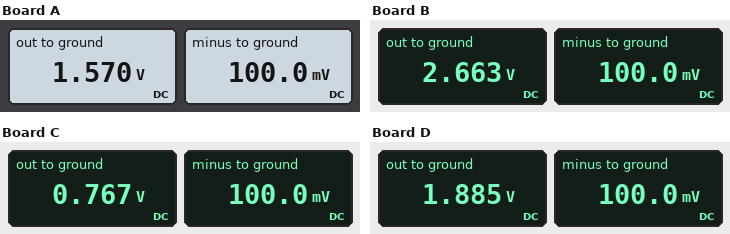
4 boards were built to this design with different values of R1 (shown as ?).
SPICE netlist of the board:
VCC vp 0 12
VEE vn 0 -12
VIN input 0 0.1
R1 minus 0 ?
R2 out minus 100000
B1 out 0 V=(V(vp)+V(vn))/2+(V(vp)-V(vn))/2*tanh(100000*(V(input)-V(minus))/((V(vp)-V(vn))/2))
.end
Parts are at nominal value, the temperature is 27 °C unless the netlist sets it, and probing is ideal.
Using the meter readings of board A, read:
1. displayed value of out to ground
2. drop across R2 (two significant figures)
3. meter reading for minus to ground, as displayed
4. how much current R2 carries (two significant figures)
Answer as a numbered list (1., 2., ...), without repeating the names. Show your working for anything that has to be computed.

1. 1.570 V
2. 1.57 V - 100 mV = 1.5 V
3. 100.0 mV
4. (1.57 V - 100 mV) / 100 kΩ = 15 µA
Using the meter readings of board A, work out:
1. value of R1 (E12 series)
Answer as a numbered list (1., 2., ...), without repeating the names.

1. 6.8 kΩ
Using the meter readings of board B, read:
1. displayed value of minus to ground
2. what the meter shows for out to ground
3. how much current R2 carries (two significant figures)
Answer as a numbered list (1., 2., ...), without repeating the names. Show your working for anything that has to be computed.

1. 100.0 mV
2. 2.663 V
3. (2.663 V - 100 mV) / 100 kΩ = 26 µA
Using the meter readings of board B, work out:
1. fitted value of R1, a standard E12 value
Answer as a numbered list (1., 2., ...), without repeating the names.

1. 3.9 kΩ
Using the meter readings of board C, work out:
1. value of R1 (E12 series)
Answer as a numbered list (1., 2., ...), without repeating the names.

1. 15 kΩ
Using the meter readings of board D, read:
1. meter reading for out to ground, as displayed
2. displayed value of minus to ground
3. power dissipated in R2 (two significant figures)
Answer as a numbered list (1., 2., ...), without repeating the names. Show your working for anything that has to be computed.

1. 1.885 V
2. 100.0 mV
3. (1.885 V - 100 mV)^2 / 100 kΩ = 32 µW
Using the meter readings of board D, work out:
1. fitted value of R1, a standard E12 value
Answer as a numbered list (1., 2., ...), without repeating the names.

1. 5.6 kΩ
